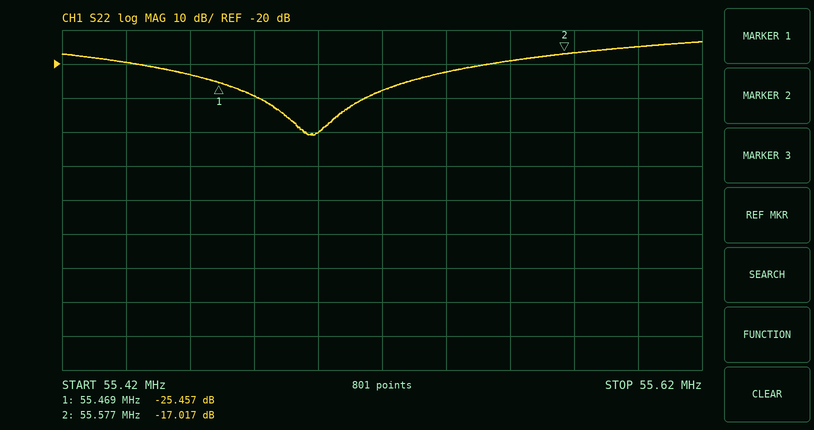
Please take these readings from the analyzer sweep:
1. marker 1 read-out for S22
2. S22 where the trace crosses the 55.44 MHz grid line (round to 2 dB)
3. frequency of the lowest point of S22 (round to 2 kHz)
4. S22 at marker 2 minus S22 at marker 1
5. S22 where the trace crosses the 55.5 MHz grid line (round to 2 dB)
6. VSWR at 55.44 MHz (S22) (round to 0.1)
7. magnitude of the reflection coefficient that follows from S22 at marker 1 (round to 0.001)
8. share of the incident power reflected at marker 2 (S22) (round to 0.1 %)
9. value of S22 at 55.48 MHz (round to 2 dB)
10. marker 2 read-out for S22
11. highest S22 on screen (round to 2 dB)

-25.457 dB
-20 dB
55.498 MHz
8.440 dB
-40 dB
1.2
0.053
2.0 %
-30 dB
-17.017 dB
-14 dB
